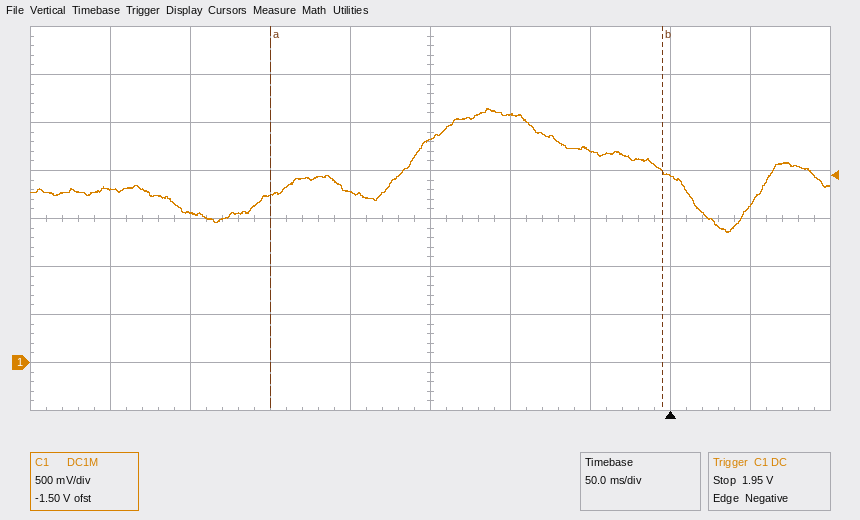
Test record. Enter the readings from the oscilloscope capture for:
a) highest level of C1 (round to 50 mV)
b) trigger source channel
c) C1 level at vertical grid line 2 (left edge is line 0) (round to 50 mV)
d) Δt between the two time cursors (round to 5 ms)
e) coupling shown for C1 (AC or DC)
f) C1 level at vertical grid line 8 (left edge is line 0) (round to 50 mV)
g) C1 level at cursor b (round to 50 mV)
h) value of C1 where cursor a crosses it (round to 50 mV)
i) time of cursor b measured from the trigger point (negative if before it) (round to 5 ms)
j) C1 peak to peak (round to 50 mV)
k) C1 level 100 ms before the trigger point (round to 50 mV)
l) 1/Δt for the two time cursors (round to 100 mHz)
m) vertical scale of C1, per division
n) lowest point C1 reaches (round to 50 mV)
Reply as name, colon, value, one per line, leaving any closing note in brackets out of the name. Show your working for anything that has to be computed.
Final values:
highest level of C1: 2.65 V
trigger source channel: C1
C1 level at vertical grid line 2 (left edge is line 0): 1.55 V
Δt between the two time cursors: 245 ms
coupling shown for C1: DC
C1 level at vertical grid line 8 (left edge is line 0): 1.95 V
C1 level at cursor b: 2.00 V
value of C1 where cursor a crosses it: 1.75 V
time of cursor b measured from the trigger point (negative if before it): -5 ms
C1 peak to peak: 2.65 V − (1.35 V) = 1.30 V
C1 level 100 ms before the trigger point: 2.60 V
1/Δt for the two time cursors: 1 / 245 ms ≈ 4.1 Hz
vertical scale of C1, per division: 500 mV
lowest point C1 reaches: 1.35 V
